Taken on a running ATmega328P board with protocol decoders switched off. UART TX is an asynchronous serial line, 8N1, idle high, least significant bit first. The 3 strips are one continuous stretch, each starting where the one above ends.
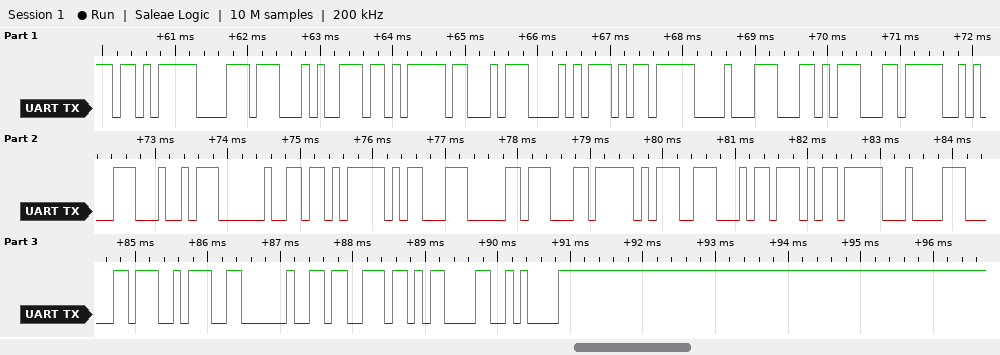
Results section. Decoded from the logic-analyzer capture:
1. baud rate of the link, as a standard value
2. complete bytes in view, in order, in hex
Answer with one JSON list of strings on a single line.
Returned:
["9600 baud", "EB B8 94 EB A3 A8 ED 88 AC EC 8A A4 20 EB 8D B0 EC 9D B4 ED 84 B0 3A 20 73 0D 0A"]
